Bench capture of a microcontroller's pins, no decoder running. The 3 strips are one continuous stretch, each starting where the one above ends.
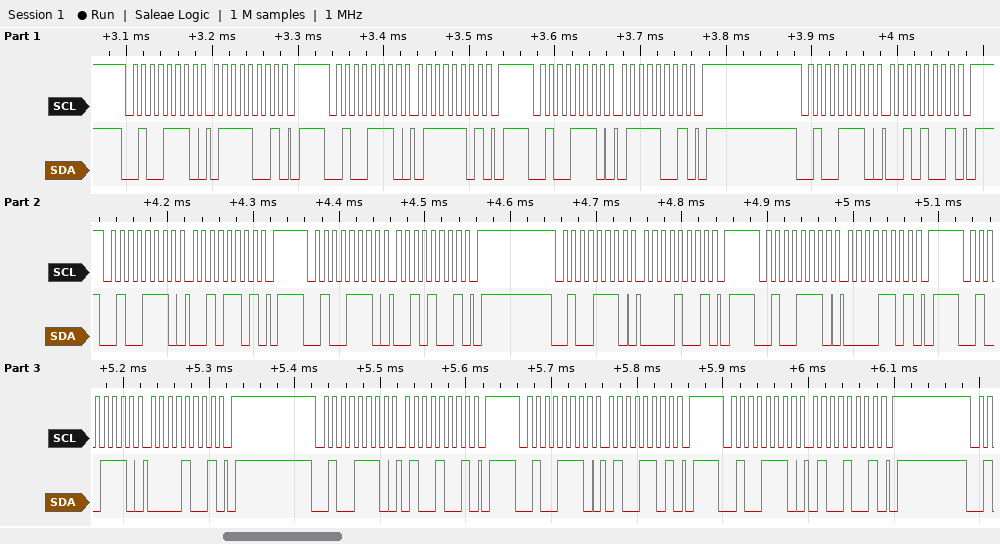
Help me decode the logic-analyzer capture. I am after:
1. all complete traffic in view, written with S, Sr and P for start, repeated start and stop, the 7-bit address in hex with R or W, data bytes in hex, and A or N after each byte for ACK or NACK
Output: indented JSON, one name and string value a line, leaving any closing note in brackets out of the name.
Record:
{
  "all complete traffic in view, written with S, Sr and P for start, repeated start and stop, the 7-bit address in hex with R or W, data bytes in hex, and A or N after each byte for ACK or NACK": "S 27W A 79 A P S 27W A 7D A P S 27W A 79 A P S 27W A 29 A P S 27W A 2D A P S 27W A 29 A P S 27W A 09 A P S 27W A 0D A P S 27W A 09 A P S 27W A 49 A P S 27W A 4D A P S 27W A 49 A P"
}
